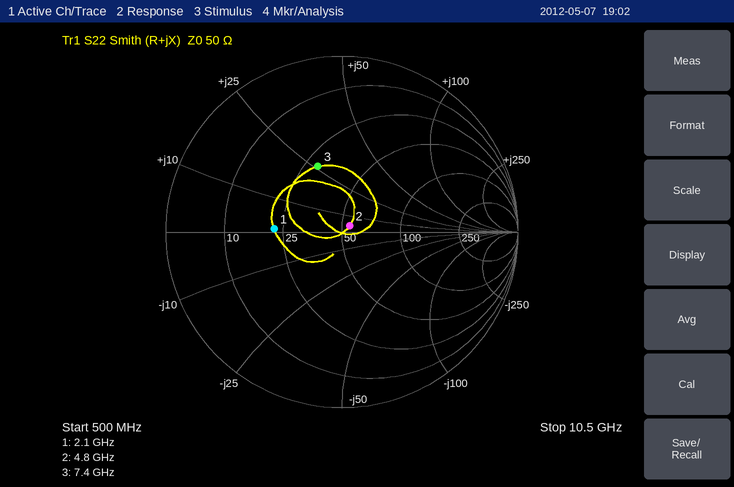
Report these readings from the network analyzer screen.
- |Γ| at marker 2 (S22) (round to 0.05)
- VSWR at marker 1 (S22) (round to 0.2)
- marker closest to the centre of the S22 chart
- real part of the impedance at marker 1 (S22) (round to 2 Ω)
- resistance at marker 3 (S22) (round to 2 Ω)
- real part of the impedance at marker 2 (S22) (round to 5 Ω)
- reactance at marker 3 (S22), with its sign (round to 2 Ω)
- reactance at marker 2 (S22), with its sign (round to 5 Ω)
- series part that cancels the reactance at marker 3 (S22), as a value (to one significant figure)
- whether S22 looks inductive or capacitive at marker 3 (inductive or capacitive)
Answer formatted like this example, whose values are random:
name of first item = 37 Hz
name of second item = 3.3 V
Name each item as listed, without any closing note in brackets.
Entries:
|Γ| at marker 2 (S22) = 0.05
VSWR at marker 1 (S22) = 2.2
marker closest to the centre of the S22 chart = marker 2
real part of the impedance at marker 1 (S22) = 22 Ω
resistance at marker 3 (S22) = 30 Ω
real part of the impedance at marker 2 (S22) = 55 Ω
reactance at marker 3 (S22), with its sign = +26 Ω
reactance at marker 2 (S22), with its sign = +5 Ω
series part that cancels the reactance at marker 3 (S22), as a value = 800 fF
whether S22 looks inductive or capacitive at marker 3 = inductive
